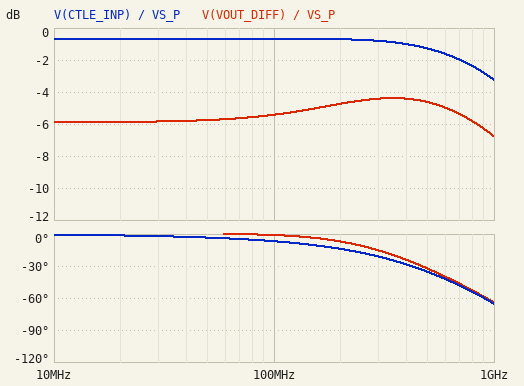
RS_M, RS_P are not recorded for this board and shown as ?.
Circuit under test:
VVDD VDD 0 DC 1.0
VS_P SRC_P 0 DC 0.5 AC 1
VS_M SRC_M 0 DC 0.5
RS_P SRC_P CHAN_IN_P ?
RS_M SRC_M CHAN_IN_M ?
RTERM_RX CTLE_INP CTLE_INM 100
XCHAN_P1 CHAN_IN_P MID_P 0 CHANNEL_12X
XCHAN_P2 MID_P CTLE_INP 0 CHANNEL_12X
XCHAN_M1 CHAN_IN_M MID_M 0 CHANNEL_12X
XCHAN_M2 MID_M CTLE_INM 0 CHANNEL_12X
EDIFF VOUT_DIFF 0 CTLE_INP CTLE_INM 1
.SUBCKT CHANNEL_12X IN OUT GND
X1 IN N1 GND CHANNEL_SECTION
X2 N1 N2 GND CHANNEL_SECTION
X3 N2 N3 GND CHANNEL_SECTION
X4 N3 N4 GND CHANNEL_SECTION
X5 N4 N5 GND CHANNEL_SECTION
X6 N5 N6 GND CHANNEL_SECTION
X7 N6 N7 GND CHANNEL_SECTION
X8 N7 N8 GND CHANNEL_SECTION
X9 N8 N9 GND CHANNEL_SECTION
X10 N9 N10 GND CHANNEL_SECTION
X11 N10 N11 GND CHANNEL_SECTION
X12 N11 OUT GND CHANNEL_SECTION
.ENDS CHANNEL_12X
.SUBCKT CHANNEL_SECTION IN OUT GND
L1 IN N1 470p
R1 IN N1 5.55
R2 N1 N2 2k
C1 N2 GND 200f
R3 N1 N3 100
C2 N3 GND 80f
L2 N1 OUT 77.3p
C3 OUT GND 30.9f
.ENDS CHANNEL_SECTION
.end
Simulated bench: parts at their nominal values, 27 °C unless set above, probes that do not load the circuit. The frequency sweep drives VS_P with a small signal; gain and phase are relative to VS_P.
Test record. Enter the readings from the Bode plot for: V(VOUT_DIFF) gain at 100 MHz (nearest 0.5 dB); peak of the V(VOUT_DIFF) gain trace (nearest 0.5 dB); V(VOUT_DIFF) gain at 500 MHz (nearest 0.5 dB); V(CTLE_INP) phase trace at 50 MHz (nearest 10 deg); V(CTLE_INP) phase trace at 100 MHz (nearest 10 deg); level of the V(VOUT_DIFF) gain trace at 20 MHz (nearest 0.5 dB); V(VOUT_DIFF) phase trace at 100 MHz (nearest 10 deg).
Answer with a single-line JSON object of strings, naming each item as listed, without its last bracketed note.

{"V(VOUT_DIFF) gain at 100 MHz": "-5.5 dB", "peak of the V(VOUT_DIFF) gain trace": "-4.5 dB", "V(VOUT_DIFF) gain at 500 MHz": "-4.5 dB", "V(CTLE_INP) phase trace at 50 MHz": "0 deg", "V(CTLE_INP) phase trace at 100 MHz": "-10 deg", "level of the V(VOUT_DIFF) gain trace at 20 MHz": "-6.0 dB", "V(VOUT_DIFF) phase trace at 100 MHz": "0 deg"}
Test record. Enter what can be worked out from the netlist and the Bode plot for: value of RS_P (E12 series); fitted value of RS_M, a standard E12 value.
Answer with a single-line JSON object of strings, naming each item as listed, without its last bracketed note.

{"value of RS_P": "15 Ω", "fitted value of RS_M, a standard E12 value": "82 Ω"}
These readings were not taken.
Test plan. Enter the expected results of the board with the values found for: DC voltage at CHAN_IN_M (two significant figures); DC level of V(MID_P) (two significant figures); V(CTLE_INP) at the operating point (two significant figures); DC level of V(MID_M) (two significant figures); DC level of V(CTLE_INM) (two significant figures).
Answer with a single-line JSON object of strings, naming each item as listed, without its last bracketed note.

{"DC voltage at CHAN_IN_M": "500 mV", "DC level of V(MID_P)": "500 mV", "V(CTLE_INP) at the operating point": "500 mV", "DC level of V(MID_M)": "500 mV", "DC level of V(CTLE_INM)": "500 mV"}
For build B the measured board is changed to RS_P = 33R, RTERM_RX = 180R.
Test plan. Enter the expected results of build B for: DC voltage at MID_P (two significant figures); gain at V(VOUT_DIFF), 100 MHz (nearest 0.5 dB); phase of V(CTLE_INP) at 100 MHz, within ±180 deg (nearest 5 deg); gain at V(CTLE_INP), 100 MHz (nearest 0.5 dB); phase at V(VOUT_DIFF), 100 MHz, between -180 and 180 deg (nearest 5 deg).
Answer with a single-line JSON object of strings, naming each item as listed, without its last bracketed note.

{"DC voltage at MID_P": "500 mV", "gain at V(VOUT_DIFF), 100 MHz": "-4.0 dB", "phase of V(CTLE_INP) at 100 MHz, within ±180 deg": "-10 deg", "gain at V(CTLE_INP), 100 MHz": "-1.0 dB", "phase at V(VOUT_DIFF), 100 MHz, between -180 and 180 deg": "-5 deg"}
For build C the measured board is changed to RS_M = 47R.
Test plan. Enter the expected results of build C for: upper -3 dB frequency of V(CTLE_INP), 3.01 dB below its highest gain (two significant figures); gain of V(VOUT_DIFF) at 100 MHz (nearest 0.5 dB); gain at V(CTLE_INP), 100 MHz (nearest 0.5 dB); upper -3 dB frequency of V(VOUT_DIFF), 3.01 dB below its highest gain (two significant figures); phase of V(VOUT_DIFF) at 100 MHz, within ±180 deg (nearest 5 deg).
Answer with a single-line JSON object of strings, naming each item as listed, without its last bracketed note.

{"upper -3 dB frequency of V(CTLE_INP), 3.01 dB below its highest gain": "1.2 GHz", "gain of V(VOUT_DIFF) at 100 MHz": "-4.0 dB", "gain at V(CTLE_INP), 100 MHz": "-1.0 dB", "upper -3 dB frequency of V(VOUT_DIFF), 3.01 dB below its highest gain": "990 MHz", "phase of V(VOUT_DIFF) at 100 MHz, within ±180 deg": "-5 deg"}
